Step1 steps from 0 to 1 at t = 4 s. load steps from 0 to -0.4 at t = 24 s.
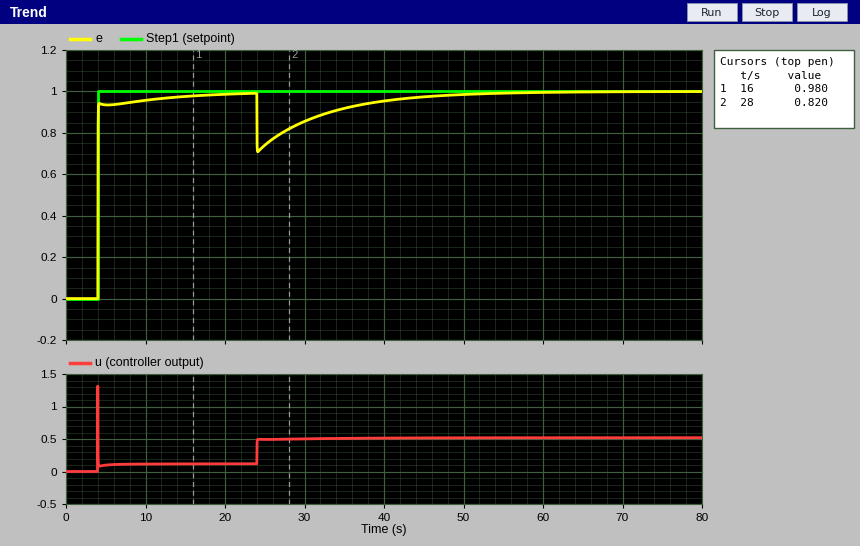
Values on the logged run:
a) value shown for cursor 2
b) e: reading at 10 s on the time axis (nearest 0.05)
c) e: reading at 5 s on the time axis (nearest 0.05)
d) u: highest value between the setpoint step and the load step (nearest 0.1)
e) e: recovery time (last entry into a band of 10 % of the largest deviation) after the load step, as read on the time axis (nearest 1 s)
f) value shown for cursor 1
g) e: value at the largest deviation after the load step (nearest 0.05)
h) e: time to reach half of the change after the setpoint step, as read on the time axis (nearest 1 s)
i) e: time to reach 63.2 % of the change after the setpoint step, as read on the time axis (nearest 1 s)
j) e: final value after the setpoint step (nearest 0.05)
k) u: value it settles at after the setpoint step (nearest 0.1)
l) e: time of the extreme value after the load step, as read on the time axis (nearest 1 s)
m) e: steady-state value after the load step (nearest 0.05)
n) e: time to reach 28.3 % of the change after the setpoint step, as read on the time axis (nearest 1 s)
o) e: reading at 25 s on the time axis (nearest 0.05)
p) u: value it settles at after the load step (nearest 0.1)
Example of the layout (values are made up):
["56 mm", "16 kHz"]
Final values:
["0.820", "0.95", "0.95", "1.3", "44 s", "0.980", "0.70", "4 s", "4 s", "1.00", "0.1", "24 s", "1.00", "4 s", "0.75", "0.5"]
